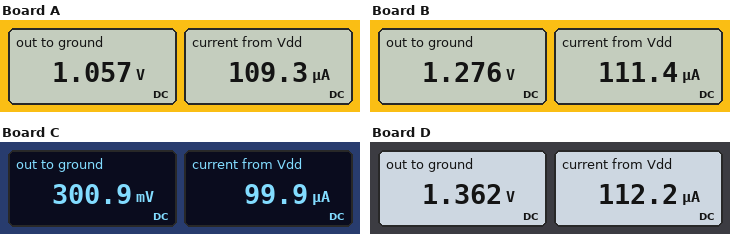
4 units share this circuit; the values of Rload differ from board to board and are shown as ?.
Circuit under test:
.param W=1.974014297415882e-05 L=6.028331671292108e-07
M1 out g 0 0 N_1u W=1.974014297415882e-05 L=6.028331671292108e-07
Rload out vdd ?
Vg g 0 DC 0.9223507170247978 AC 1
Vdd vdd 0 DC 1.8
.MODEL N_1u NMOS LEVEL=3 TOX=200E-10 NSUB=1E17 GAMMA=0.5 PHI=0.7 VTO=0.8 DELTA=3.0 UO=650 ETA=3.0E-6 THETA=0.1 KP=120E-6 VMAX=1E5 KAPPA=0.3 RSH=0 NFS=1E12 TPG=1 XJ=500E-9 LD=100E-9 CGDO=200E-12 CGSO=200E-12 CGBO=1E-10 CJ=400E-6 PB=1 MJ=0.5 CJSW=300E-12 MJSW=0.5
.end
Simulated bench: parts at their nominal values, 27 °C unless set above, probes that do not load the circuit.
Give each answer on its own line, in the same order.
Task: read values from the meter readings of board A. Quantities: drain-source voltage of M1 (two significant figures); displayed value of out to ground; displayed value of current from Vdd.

1.1 V
1.057 V
109.3 µA
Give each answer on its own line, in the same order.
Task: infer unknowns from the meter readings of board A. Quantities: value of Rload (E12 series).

6.8 kΩ
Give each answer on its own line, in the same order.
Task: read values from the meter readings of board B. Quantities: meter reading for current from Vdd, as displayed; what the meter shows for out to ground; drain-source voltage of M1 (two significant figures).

111.4 µA
1.276 V
1.3 V
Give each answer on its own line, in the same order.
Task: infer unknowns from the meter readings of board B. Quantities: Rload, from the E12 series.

4.7 kΩ
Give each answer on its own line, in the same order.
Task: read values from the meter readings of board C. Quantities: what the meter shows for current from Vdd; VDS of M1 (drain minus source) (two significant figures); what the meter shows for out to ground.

99.9 µA
300 mV
300.9 mV
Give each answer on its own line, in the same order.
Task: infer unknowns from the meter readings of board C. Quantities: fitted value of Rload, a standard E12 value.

15 kΩ
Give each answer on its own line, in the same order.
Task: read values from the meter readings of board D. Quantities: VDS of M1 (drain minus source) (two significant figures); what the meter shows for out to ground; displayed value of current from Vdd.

1.4 V
1.362 V
112.2 µA
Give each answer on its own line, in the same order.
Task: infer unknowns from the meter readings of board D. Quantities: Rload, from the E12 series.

3.9 kΩ
